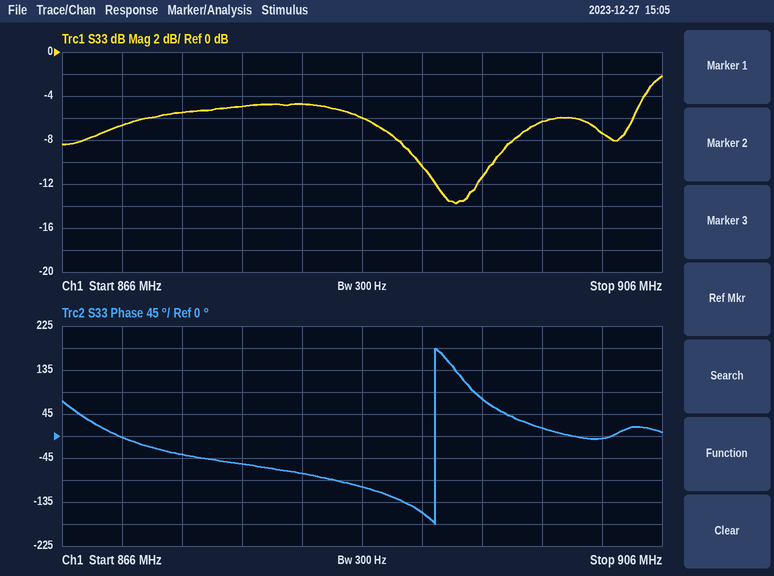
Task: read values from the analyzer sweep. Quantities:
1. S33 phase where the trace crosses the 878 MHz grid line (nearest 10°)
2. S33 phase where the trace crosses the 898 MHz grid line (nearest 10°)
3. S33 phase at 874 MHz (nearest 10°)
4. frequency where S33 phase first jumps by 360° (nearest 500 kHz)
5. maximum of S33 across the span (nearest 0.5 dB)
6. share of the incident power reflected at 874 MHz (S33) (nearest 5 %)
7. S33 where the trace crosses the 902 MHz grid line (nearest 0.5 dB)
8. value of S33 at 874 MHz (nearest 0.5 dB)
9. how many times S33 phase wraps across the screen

-60°
20°
-40°
891.0 MHz
-2.0 dB
30 %
-7.5 dB
-5.5 dB
1
